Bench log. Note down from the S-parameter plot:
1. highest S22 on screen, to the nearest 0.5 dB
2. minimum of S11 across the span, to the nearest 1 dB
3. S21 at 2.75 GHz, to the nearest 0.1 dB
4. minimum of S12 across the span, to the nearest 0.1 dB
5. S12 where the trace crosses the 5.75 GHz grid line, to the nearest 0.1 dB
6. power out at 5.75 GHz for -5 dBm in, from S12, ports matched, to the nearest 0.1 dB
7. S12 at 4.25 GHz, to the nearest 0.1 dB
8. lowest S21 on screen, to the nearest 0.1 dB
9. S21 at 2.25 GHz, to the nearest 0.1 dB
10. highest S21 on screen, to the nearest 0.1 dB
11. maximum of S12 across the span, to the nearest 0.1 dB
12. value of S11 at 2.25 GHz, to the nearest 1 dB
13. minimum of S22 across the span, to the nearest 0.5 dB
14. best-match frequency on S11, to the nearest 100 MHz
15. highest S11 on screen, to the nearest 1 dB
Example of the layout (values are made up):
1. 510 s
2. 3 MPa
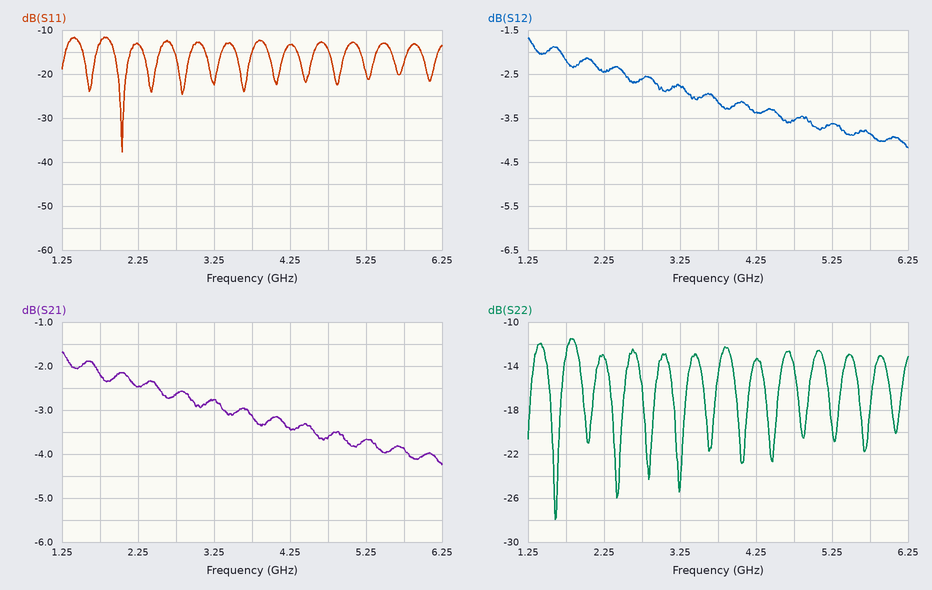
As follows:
1. -11.5 dB
2. -38 dB
3. -2.6 dB
4. -4.2 dB
5. -3.9 dB
6. -8.9 dBm
7. -3.4 dB
8. -4.2 dB
9. -2.5 dB
10. -1.7 dB
11. -1.7 dB
12. -13 dB
13. -28.0 dB
14. 2.0 GHz
15. -12 dB
